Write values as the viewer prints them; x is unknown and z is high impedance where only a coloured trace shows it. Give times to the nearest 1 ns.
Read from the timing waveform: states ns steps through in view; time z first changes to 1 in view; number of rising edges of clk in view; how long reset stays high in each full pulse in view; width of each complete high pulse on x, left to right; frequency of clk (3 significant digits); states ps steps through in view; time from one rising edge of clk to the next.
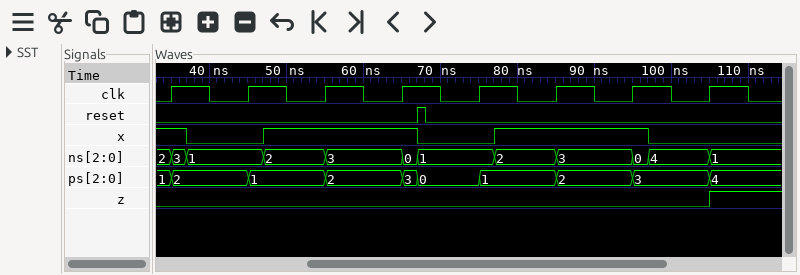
2, 3, 1, 2, 3, 0, 1, 2, 3, 0, 4, 1
105 ns
8
1 ns
20 ns, 20 ns
100 MHz
1, 2, 1, 2, 3, 0, 1, 2, 3, 4
10 ns
